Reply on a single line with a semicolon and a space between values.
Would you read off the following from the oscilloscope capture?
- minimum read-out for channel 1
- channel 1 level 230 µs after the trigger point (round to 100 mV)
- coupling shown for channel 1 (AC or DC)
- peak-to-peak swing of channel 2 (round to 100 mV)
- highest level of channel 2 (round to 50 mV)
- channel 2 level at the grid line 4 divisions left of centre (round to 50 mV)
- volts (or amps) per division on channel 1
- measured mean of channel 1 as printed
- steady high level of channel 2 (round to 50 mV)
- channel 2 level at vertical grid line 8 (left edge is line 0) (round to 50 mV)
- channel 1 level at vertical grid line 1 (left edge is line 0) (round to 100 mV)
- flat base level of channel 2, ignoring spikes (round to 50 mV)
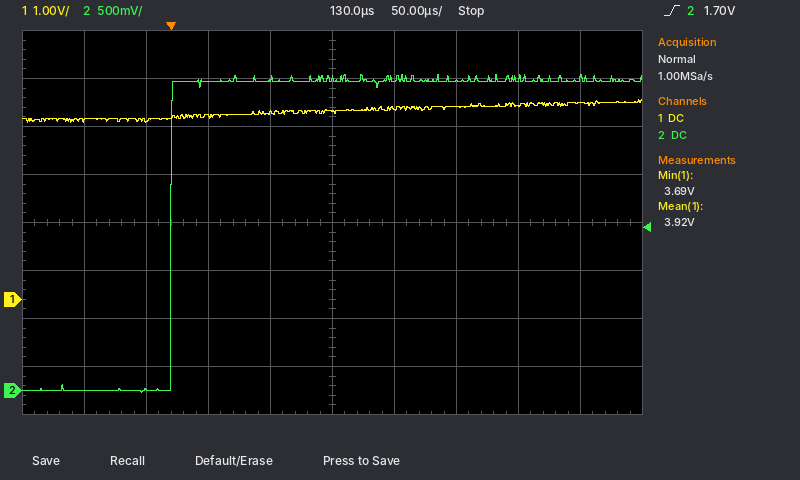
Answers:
3.69 V; 4.0 V; DC; 3.30 V; 3.30 V; 0 mV; 1 V; 3.92 V; 3.20 V; 3.25 V; 3.7 V; 0 mV
